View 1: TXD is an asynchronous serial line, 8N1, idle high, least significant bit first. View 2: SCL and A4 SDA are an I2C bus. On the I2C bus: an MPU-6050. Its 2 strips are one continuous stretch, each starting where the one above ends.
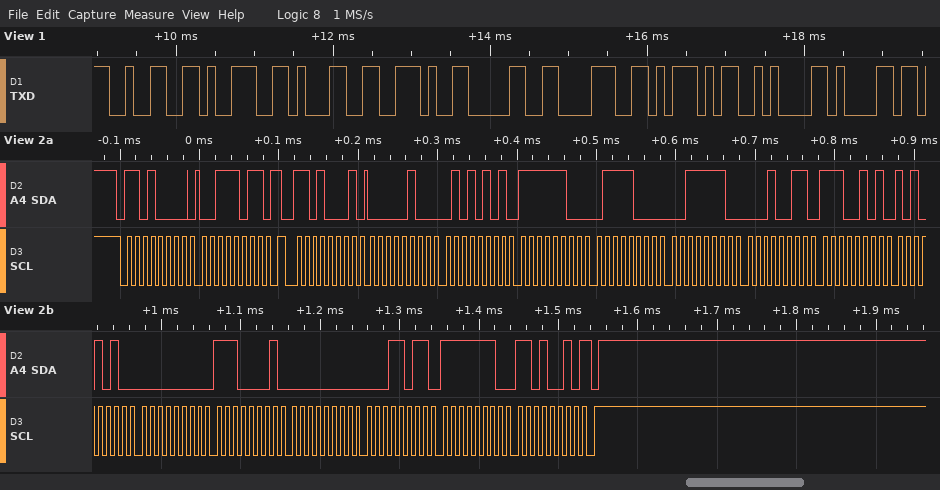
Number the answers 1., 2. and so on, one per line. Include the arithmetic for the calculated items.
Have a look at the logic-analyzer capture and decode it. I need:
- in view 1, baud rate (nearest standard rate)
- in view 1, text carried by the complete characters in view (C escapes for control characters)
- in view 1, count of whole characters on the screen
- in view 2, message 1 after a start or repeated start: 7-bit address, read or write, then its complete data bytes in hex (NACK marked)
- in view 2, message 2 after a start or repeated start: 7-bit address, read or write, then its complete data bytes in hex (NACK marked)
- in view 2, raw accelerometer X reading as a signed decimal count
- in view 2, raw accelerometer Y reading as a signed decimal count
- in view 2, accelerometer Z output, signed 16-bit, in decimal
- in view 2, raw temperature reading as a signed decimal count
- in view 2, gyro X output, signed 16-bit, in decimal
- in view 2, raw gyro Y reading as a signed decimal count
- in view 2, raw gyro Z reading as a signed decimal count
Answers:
1. 9600 baud
2. "291.08]\na"
3. 9
4. 0x68 write: 3B
5. 0x68 read: 04 55 FC 78 3E 13 E5 AA 00 E1 00 1B FE D2 NACK
6. 0x0455 = 1109
7. 0xFC78 = -904
8. 0x3E13 = 15891
9. 0xE5AA = -6742
10. 0x00E1 = 225
11. 0x001B = 27
12. 0xFED2 = -302
